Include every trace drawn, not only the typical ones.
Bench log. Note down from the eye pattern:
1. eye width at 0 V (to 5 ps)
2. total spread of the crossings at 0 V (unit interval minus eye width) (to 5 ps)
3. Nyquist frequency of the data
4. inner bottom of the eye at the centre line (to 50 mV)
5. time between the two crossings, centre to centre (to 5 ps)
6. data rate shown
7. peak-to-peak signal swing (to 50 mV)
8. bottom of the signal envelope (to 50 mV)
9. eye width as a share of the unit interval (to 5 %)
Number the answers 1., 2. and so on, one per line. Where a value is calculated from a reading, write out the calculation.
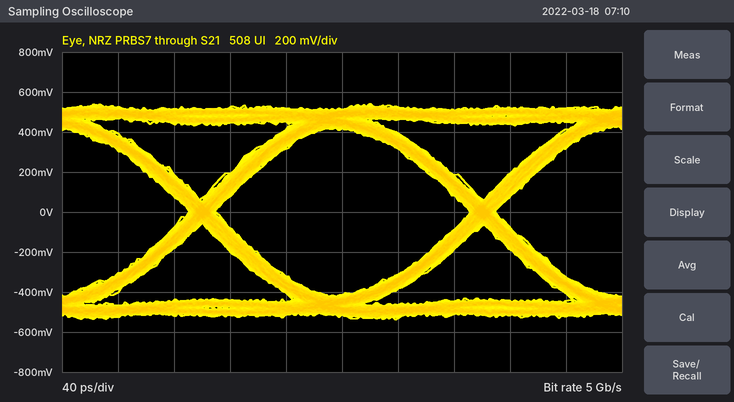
1. 180 ps
2. 20 ps
3. 2.5 GHz
4. -400 mV
5. 200 ps
6. 5 Gb/s
7. 1.10 V
8. -550 mV
9. 180 ps / 200 ps ≈ 90 %
